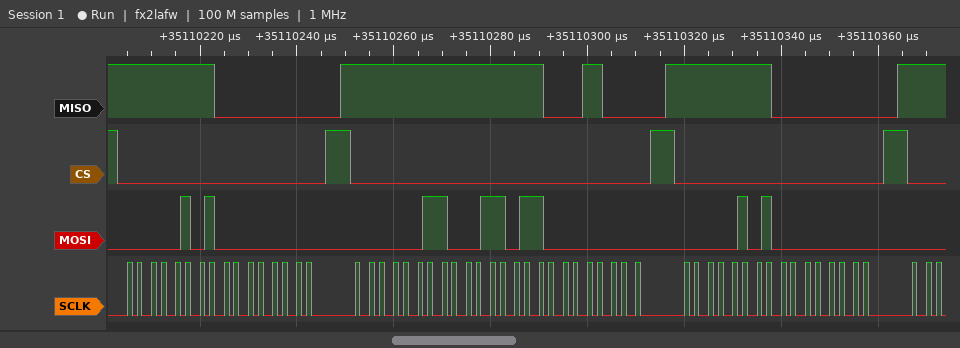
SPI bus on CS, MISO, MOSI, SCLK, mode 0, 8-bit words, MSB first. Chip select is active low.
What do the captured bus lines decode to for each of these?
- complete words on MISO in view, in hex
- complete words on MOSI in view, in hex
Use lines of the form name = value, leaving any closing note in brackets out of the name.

complete words on MISO in view, in hex = FF, 00, FF, FF, 18, FF, 00
complete words on MOSI in view, in hex = 05, 00, 03, 1B, 00, 05, 00
